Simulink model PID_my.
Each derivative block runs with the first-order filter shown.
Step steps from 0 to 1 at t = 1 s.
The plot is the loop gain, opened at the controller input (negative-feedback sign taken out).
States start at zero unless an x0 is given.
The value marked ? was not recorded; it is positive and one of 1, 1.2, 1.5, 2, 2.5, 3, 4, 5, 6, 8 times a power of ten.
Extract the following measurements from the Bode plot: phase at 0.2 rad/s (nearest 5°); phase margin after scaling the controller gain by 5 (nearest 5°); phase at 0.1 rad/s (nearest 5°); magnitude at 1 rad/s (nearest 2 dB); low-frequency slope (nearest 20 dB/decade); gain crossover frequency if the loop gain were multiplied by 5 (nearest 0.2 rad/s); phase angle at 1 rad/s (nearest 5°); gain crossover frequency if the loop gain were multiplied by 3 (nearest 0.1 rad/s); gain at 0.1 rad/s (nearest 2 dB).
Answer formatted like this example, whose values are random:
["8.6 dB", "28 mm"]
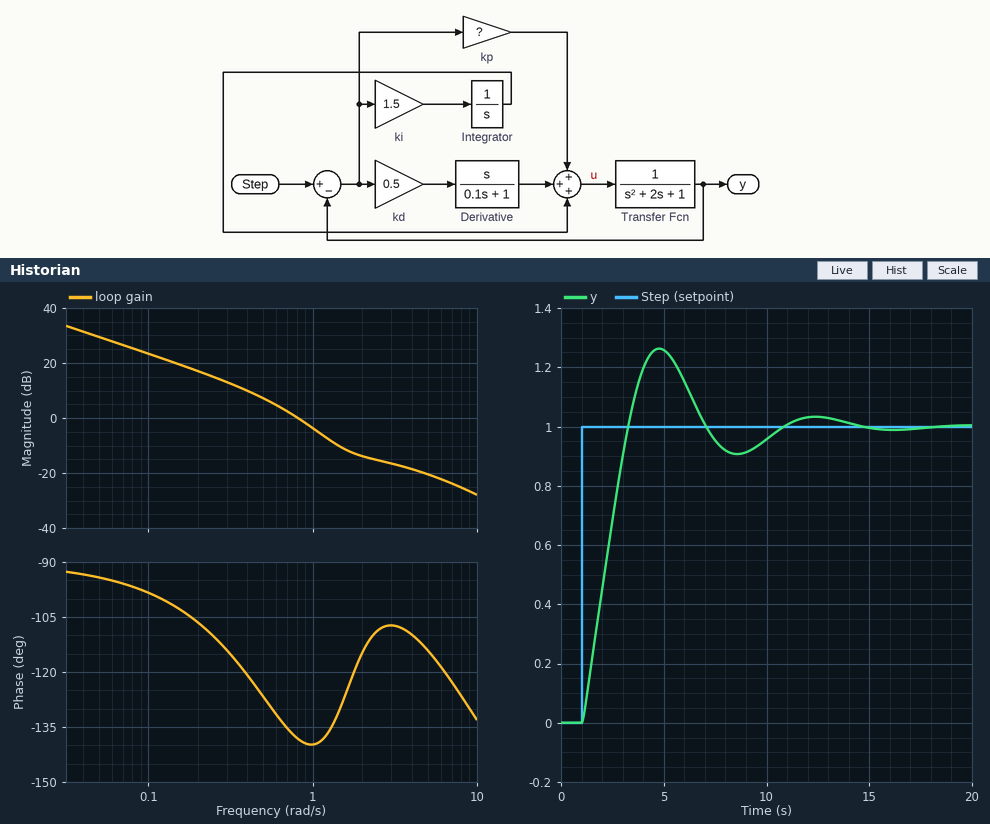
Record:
["-105°", "65°", "-100°", "-4 dB", "-20 dB/decade", "2.0 rad/s", "-140°", "1.4 rad/s", "24 dB"]
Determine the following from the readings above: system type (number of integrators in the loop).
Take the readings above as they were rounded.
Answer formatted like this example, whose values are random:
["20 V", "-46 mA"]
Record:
["1"]
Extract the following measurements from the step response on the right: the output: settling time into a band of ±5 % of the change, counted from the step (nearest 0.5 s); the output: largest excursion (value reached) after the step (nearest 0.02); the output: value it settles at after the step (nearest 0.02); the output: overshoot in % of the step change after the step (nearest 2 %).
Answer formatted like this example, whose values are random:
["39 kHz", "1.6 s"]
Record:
["9.0 s", "1.26", "1.00", "26 %"]
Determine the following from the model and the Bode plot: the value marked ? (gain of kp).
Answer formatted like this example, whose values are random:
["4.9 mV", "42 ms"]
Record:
["0.8"]
